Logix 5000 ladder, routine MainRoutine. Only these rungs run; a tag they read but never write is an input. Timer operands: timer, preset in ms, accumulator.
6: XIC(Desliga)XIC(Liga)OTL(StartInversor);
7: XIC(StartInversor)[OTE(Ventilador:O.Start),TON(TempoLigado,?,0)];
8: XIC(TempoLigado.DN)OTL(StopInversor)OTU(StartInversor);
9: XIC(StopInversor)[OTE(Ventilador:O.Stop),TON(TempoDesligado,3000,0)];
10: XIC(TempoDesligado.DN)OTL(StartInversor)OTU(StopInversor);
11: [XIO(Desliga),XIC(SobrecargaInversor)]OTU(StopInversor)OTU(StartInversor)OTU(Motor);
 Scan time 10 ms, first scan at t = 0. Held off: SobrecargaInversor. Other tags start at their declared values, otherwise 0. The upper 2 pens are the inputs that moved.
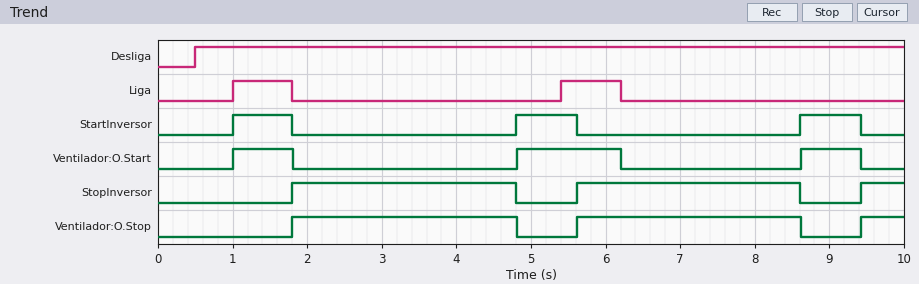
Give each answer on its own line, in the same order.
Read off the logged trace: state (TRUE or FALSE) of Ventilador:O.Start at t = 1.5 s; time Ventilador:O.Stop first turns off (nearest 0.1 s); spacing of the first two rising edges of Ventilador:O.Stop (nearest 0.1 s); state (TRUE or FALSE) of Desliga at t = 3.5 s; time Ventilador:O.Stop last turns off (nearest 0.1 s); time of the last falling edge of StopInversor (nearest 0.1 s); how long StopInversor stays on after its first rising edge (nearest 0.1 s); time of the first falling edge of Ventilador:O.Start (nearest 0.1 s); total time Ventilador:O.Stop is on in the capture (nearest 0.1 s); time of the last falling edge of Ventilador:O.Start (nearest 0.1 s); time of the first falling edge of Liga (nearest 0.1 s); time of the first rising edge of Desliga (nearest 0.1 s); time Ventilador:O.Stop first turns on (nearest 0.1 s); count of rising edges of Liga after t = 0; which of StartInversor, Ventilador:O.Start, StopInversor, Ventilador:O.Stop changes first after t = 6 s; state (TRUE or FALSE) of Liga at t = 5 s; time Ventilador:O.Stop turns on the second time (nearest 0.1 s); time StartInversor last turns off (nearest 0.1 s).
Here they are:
TRUE
4.8 s
3.8 s
TRUE
8.6 s
8.6 s
3.0 s
1.8 s
6.6 s
9.4 s
1.8 s
0.5 s
1.8 s
2
Ventilador:O.Start
FALSE
5.6 s
9.4 s
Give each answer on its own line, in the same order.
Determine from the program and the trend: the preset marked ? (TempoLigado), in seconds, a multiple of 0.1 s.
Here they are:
0.8 s
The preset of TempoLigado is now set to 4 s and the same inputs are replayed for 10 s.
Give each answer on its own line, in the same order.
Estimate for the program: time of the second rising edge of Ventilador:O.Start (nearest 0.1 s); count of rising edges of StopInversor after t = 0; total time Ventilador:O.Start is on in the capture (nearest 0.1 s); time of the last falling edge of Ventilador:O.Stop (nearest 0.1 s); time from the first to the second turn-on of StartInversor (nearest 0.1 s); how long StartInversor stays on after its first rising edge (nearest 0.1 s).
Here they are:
5.4 s
2
8.0 s
8.0 s
4.4 s
4.0 s
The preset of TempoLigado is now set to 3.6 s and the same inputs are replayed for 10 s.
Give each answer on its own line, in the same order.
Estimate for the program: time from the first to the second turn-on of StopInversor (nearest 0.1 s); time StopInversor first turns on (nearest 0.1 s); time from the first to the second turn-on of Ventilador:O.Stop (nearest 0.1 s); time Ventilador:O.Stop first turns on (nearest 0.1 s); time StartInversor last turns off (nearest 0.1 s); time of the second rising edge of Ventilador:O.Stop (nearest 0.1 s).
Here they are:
4.4 s
4.6 s
4.4 s
4.6 s
9.0 s
9.0 s
